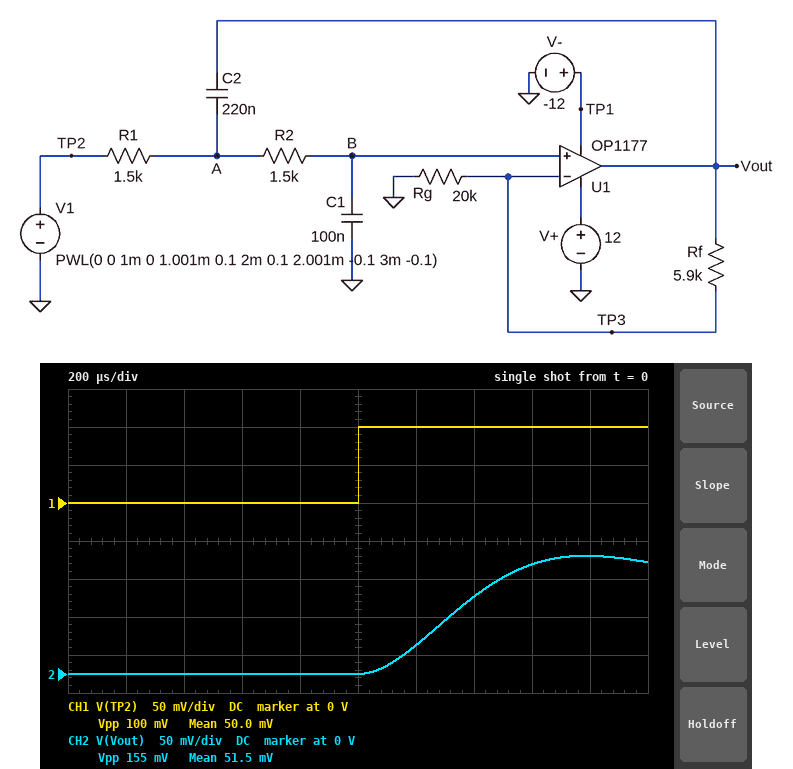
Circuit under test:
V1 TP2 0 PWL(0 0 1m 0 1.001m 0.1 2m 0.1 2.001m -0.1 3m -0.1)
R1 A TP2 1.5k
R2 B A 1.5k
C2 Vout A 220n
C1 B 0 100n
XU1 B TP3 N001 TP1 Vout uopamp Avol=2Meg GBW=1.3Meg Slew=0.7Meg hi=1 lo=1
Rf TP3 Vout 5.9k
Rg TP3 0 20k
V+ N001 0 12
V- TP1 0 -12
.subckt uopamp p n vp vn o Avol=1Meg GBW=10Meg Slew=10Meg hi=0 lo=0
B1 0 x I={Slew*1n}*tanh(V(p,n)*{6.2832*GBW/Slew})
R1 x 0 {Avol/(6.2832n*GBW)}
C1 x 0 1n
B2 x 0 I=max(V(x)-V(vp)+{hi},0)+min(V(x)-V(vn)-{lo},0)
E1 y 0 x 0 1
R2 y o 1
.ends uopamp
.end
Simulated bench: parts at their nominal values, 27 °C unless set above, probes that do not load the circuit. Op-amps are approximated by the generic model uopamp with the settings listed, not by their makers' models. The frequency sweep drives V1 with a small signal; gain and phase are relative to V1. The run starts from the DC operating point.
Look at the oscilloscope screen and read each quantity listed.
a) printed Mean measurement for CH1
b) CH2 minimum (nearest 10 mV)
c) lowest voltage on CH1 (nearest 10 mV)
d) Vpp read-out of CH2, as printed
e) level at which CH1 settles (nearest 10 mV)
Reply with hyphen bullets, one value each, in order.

- 50.0 mV
- 0 V
- 0 V
- 155 mV
- 100 mV
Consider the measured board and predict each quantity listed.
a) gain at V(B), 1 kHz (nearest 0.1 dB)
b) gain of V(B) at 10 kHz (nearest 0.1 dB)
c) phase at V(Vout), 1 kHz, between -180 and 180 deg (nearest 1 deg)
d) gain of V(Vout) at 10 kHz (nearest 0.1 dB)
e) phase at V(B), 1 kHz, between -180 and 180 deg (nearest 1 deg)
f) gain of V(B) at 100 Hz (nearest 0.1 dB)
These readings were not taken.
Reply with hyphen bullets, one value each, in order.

- -4.0 dB
- -45.8 dB
- -127 deg
- -43.6 dB
- -127 deg
- 0.1 dB
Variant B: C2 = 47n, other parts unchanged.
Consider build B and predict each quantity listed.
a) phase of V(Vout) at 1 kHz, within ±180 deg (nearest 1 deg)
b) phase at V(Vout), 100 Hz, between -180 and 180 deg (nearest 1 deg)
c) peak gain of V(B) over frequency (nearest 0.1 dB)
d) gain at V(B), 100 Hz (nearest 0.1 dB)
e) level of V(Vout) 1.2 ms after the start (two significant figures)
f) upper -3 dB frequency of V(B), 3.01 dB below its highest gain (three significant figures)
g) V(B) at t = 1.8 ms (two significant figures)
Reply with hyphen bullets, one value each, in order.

- -72 deg
- -10 deg
- 0 dB
- -0.1 dB
- 61 mV
- 657 Hz
- 96 mV
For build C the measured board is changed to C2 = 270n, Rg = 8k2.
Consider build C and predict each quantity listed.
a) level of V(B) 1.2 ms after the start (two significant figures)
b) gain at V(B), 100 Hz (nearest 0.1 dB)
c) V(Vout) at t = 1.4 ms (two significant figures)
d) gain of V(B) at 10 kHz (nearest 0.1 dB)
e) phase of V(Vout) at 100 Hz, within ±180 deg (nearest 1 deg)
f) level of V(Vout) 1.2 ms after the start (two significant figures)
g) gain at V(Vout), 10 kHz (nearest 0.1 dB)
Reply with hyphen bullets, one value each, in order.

- 31 mV
- 0.2 dB
- 180 mV
- -47.6 dB
- 0 deg
- 53 mV
- -42.9 dB
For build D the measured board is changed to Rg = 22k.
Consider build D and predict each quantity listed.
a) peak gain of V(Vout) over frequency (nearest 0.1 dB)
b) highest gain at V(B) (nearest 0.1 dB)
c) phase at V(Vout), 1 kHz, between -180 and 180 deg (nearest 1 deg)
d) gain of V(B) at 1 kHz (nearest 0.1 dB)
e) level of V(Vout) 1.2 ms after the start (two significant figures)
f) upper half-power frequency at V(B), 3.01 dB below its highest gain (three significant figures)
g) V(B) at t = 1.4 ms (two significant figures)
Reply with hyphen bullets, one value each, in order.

- 3.6 dB
- 1.6 dB
- -126 deg
- -4.3 dB
- 37 mV
- 841 Hz
- 77 mV
